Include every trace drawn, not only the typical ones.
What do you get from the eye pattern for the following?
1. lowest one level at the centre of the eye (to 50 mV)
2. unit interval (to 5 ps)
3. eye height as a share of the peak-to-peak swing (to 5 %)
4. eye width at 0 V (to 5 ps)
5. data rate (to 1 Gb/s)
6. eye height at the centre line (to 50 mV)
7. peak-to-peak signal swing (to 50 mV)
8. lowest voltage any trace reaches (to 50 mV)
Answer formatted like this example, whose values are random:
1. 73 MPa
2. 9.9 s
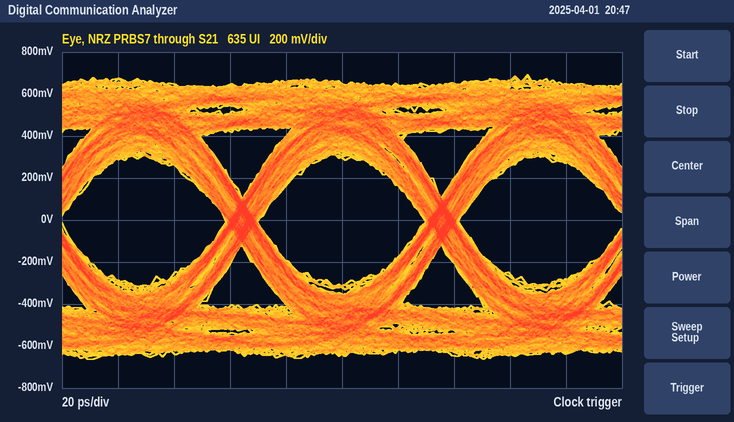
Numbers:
1. 300 mV
2. 70 ps
3. 45 %
4. 60 ps
5. 14 Gb/s
6. 600 mV
7. 1.35 V
8. -650 mV
